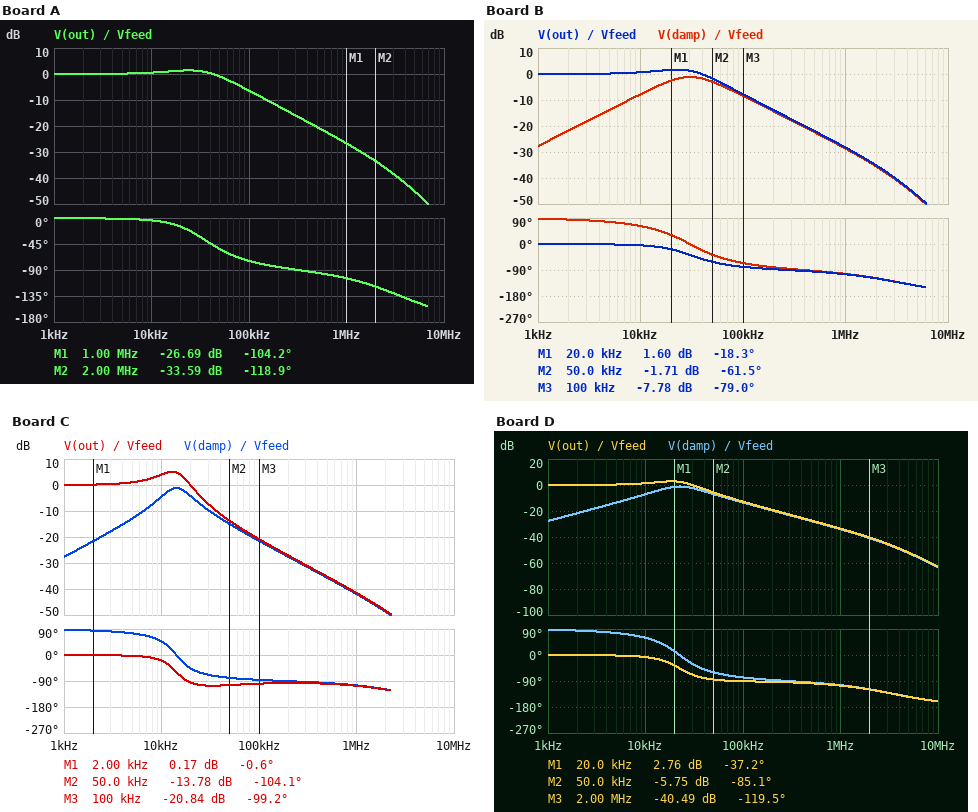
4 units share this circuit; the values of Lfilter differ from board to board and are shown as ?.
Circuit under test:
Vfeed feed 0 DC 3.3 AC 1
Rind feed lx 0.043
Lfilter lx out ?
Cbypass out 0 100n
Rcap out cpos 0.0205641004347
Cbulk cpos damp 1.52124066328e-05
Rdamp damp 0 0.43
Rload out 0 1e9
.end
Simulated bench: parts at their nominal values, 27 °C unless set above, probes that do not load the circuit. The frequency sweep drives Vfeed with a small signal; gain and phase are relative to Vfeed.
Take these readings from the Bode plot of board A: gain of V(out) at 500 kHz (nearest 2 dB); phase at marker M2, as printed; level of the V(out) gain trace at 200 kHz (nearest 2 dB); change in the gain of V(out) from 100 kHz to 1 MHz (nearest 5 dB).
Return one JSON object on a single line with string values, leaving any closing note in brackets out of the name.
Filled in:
{"gain of V(out) at 500 kHz": "-20 dB", "phase at marker M2, as printed": "-118.9 deg", "level of the V(out) gain trace at 200 kHz": "-12 dB", "change in the gain of V(out) from 100 kHz to 1 MHz": "-20 dB"}
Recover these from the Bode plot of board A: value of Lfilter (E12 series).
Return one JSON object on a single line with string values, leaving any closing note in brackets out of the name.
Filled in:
{"value of Lfilter": "1.5 µH"}
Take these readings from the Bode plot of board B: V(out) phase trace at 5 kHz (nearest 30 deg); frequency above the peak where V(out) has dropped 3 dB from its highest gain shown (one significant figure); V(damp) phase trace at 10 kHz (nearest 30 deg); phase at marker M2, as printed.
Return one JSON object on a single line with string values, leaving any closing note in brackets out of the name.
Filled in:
{"V(out) phase trace at 5 kHz": "0 deg", "frequency above the peak where V(out) has dropped 3 dB from its highest gain shown": "50 kHz", "V(damp) phase trace at 10 kHz": "60 deg", "phase at marker M2, as printed": "-61.5 deg"}
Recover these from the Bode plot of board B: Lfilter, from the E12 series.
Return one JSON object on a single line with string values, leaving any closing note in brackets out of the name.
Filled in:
{"Lfilter, from the E12 series": "1.8 µH"}
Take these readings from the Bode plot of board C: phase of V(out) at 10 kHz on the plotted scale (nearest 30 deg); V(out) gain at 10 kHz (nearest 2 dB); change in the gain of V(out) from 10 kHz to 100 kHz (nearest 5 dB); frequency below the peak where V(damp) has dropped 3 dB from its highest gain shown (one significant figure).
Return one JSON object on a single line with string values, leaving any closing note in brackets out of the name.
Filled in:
{"phase of V(out) at 10 kHz on the plotted scale": "-30 deg", "V(out) gain at 10 kHz": "4 dB", "change in the gain of V(out) from 10 kHz to 100 kHz": "-25 dB", "frequency below the peak where V(damp) has dropped 3 dB from its highest gain shown": "10 kHz"}
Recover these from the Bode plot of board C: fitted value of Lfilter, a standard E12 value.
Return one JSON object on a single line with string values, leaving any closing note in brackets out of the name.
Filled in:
{"fitted value of Lfilter, a standard E12 value": "8.2 µH"}
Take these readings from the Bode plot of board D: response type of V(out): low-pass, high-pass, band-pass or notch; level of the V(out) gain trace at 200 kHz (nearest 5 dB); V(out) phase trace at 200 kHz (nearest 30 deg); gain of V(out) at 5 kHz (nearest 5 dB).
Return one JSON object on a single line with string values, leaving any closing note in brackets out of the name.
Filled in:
{"response type of V(out): low-pass, high-pass, band-pass or notch": "low-pass", "level of the V(out) gain trace at 200 kHz": "-20 dB", "V(out) phase trace at 200 kHz": "-90 deg", "gain of V(out) at 5 kHz": "0 dB"}
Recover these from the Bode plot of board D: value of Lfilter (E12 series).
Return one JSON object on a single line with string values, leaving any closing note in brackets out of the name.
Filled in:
{"value of Lfilter": "3.3 µH"}
